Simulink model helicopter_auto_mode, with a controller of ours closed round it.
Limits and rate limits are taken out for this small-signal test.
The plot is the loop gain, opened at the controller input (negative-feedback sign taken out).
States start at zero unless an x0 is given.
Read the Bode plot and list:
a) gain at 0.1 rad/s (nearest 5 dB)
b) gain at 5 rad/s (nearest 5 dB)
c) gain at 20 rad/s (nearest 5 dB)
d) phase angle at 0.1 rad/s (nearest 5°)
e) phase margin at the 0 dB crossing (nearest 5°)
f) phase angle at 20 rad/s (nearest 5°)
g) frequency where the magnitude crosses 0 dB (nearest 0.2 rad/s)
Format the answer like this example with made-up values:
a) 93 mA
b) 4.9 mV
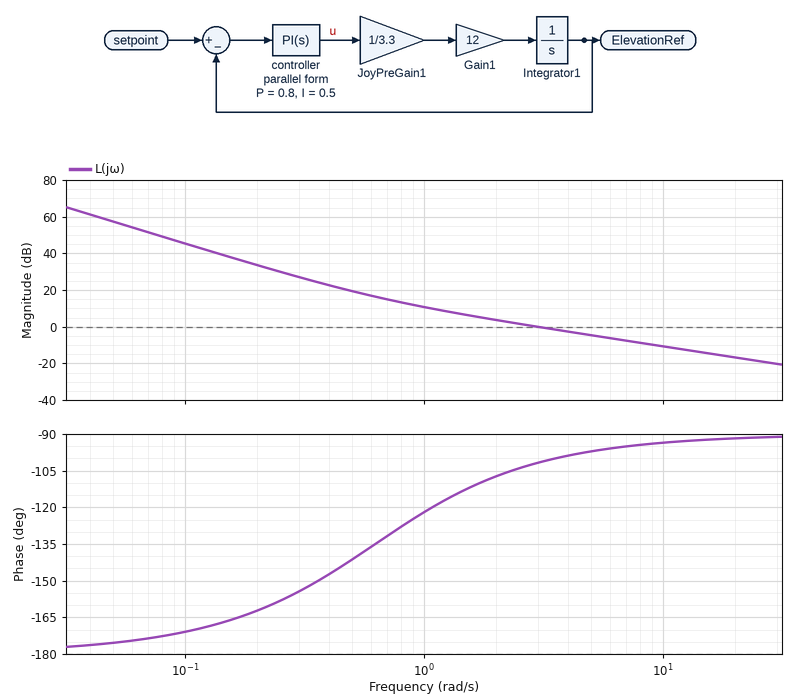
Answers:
a) 45 dB
b) -5 dB
c) -15 dB
d) -170°
e) 80°
f) -90°
g) 3.0 rad/s
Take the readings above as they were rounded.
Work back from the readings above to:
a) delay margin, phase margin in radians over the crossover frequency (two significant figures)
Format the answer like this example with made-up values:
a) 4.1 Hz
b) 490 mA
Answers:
a) 0.47 s
